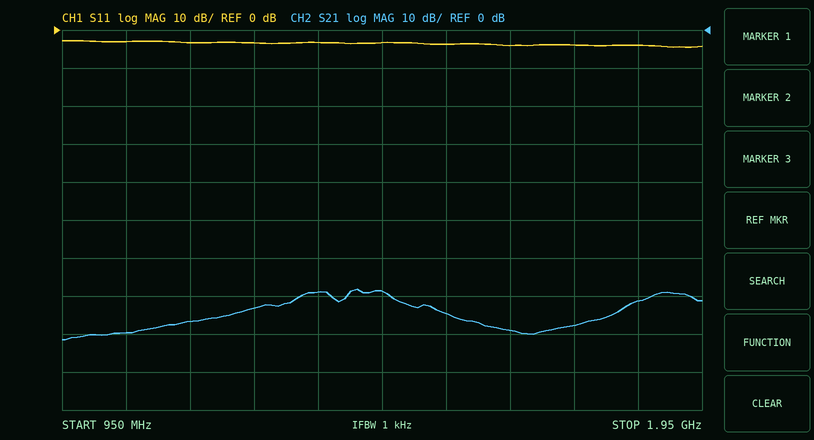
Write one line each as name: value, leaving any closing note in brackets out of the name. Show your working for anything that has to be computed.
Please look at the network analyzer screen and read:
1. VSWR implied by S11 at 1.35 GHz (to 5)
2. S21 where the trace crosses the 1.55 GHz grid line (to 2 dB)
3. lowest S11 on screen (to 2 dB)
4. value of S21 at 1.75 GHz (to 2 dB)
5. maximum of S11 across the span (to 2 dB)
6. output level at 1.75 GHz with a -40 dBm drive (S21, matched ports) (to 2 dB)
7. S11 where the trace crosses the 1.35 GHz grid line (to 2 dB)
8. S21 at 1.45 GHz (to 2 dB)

VSWR implied by S11 at 1.35 GHz: |Γ| = 10^(-4/20) = 0.6310; VSWR = (1 + 0.6310)/(1 − 0.6310) ≈ 4.42, so 5 to the nearest 5
S21 where the trace crosses the 1.55 GHz grid line: -74 dB
lowest S11 on screen: -4 dB
value of S21 at 1.75 GHz: -78 dB
maximum of S11 across the span: -2 dB
output level at 1.75 GHz with a -40 dBm drive (S21, matched ports): -40 dBm + (-78 dB) = -118 dBm
S11 where the trace crosses the 1.35 GHz grid line: -4 dB
S21 at 1.45 GHz: -68 dB
